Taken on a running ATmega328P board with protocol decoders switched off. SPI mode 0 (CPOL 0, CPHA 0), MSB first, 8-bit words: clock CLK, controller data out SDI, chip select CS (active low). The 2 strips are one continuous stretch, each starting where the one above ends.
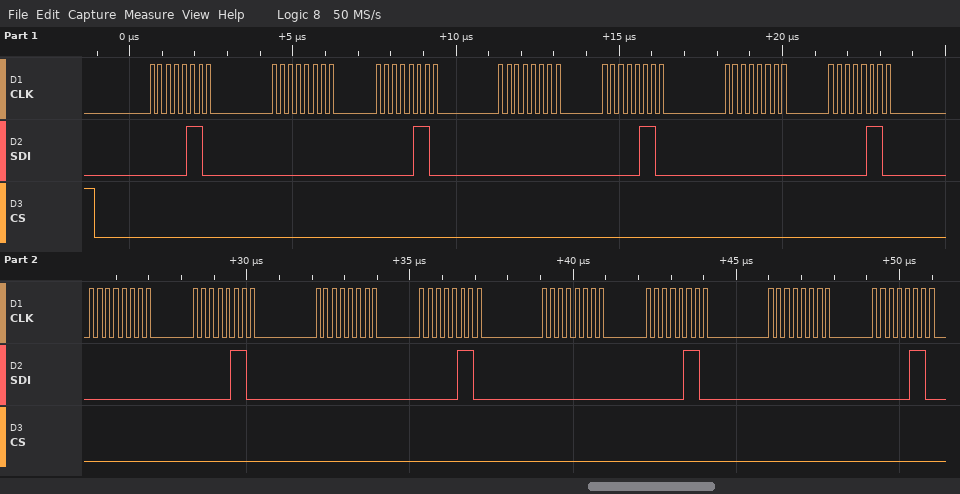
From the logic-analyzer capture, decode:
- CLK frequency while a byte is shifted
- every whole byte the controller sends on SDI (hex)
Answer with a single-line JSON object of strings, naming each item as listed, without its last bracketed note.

{"CLK frequency while a byte is shifted": "4 MHz", "every whole byte the controller sends on SDI": "06 00 06 00 06 00 06 00 06 00 06 00 06 00 06"}
